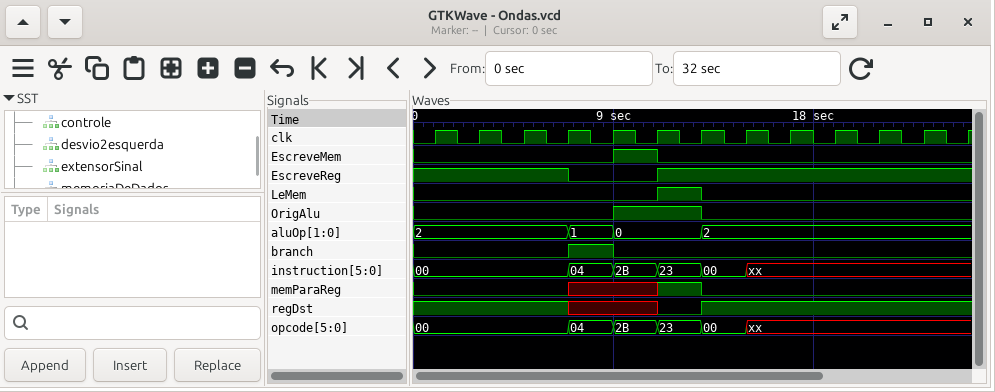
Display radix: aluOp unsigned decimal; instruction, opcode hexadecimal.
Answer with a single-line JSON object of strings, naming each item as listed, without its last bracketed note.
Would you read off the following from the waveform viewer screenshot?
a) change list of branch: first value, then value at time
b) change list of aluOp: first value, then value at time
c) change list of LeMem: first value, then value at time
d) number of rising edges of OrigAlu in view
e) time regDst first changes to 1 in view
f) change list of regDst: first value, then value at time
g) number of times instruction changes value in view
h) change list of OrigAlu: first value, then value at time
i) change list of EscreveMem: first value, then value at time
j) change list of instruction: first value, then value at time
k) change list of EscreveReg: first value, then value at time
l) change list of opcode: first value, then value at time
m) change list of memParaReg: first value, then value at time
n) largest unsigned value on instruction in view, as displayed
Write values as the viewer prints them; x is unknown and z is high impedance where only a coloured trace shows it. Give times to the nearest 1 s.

{"change list of branch: first value, then value at time": "0, 1 at 7 s, 0 at 9 s", "change list of aluOp: first value, then value at time": "2, 1 at 7 s, 0 at 9 s, 2 at 13 s", "change list of LeMem: first value, then value at time": "0, 1 at 11 s, 0 at 13 s", "number of rising edges of OrigAlu in view": "1", "time regDst first changes to 1 in view": "13 s", "change list of regDst: first value, then value at time": "1, x at 7 s, 0 at 11 s, 1 at 13 s", "number of times instruction changes value in view": "5", "change list of OrigAlu: first value, then value at time": "0, 1 at 9 s, 0 at 13 s", "change list of EscreveMem: first value, then value at time": "0, 1 at 9 s, 0 at 11 s", "change list of instruction: first value, then value at time": "00, 04 at 7 s, 2B at 9 s, 23 at 11 s, 00 at 13 s, xx at 15 s", "change list of EscreveReg: first value, then value at time": "1, 0 at 7 s, 1 at 11 s", "change list of opcode: first value, then value at time": "00, 04 at 7 s, 2B at 9 s, 23 at 11 s, 00 at 13 s, xx at 15 s", "change list of memParaReg: first value, then value at time": "0, x at 7 s, 1 at 11 s, 0 at 13 s", "largest unsigned value on instruction in view, as displayed": "2B"}
